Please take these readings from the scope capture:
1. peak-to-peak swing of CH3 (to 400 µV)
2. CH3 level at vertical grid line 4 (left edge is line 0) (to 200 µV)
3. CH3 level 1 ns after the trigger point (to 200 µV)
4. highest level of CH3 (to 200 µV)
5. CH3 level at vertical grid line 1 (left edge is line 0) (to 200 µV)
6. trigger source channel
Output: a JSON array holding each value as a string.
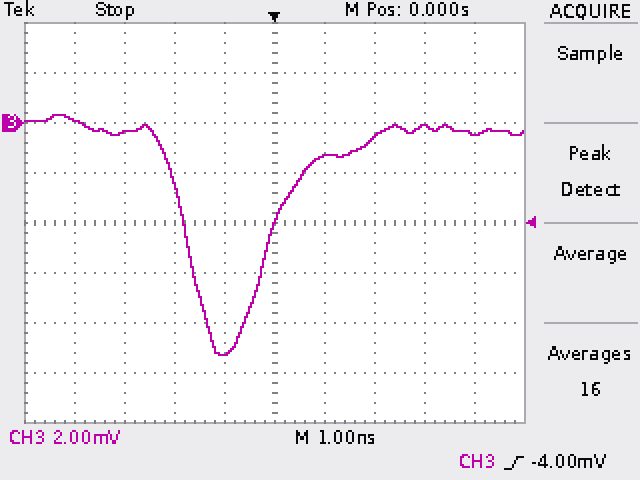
["9.6 mV", "-9.2 mV", "-1.4 mV", "400 µV", "200 µV", "CH3"]
